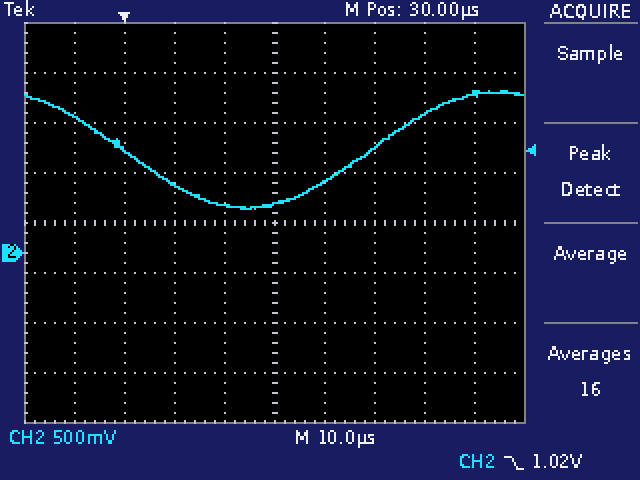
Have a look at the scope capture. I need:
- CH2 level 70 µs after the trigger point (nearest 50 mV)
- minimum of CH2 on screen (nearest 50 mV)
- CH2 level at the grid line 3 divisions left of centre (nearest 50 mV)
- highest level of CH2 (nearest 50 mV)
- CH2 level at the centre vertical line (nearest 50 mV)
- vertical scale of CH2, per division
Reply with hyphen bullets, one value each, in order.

- 1.60 V
- 450 mV
- 1.05 V
- 1.60 V
- 500 mV
- 500 mV
